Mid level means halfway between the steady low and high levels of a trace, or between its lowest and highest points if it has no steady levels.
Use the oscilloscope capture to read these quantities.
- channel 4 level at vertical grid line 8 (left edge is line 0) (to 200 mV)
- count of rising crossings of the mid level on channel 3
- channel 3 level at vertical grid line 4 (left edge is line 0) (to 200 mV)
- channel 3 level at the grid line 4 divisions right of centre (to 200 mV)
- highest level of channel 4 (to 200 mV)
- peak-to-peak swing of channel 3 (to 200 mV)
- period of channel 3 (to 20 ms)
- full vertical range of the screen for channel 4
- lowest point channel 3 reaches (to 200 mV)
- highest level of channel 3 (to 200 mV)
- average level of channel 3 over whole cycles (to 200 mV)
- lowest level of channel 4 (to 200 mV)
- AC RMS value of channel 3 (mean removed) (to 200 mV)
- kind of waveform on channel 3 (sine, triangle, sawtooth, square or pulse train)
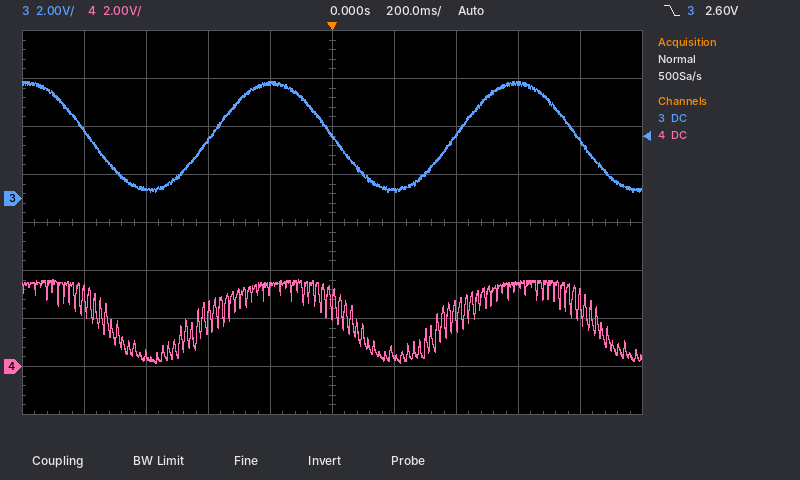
3.4 V
2
4.8 V
2.4 V
3.6 V
4.6 V
780 ms
16 V
200 mV
4.8 V
2.6 V
200 mV
1.6 V
sine
